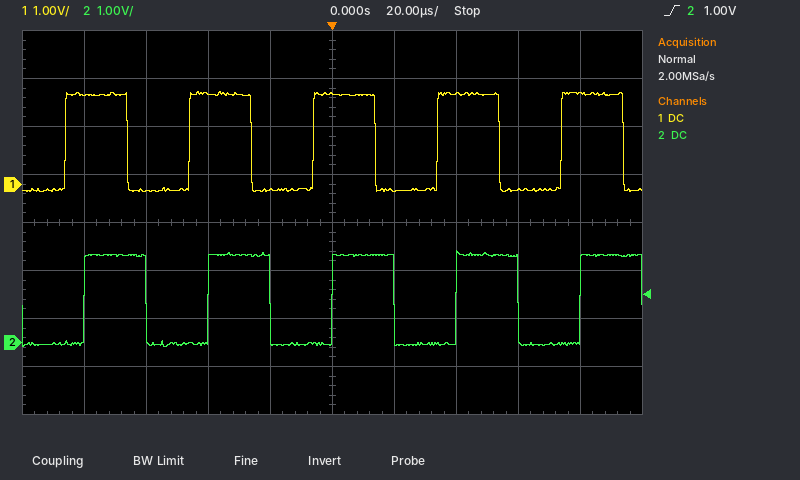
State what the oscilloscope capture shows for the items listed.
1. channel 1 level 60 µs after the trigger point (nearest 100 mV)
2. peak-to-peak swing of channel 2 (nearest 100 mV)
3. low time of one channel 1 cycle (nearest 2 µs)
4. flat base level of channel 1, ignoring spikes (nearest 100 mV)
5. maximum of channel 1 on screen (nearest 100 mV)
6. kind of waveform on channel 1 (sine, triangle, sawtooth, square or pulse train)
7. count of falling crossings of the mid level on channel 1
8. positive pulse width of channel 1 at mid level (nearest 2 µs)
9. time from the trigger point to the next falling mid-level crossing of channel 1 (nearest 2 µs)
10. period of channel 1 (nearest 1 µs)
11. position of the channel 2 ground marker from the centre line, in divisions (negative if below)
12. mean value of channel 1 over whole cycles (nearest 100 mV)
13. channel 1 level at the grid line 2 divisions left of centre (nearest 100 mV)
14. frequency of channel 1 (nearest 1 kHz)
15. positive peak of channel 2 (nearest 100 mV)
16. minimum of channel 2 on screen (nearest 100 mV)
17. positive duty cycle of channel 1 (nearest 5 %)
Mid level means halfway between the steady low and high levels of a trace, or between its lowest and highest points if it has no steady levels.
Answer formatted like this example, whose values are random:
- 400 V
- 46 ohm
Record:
- -100 mV
- 2.0 V
- 20 µs
- -100 mV
- 1.9 V
- square
- 5
- 20 µs
- 14 µs
- 40 µs
- -2.5 div
- 900 mV
- 1.9 V
- 25 kHz
- 1.9 V
- -100 mV
- 50 %
